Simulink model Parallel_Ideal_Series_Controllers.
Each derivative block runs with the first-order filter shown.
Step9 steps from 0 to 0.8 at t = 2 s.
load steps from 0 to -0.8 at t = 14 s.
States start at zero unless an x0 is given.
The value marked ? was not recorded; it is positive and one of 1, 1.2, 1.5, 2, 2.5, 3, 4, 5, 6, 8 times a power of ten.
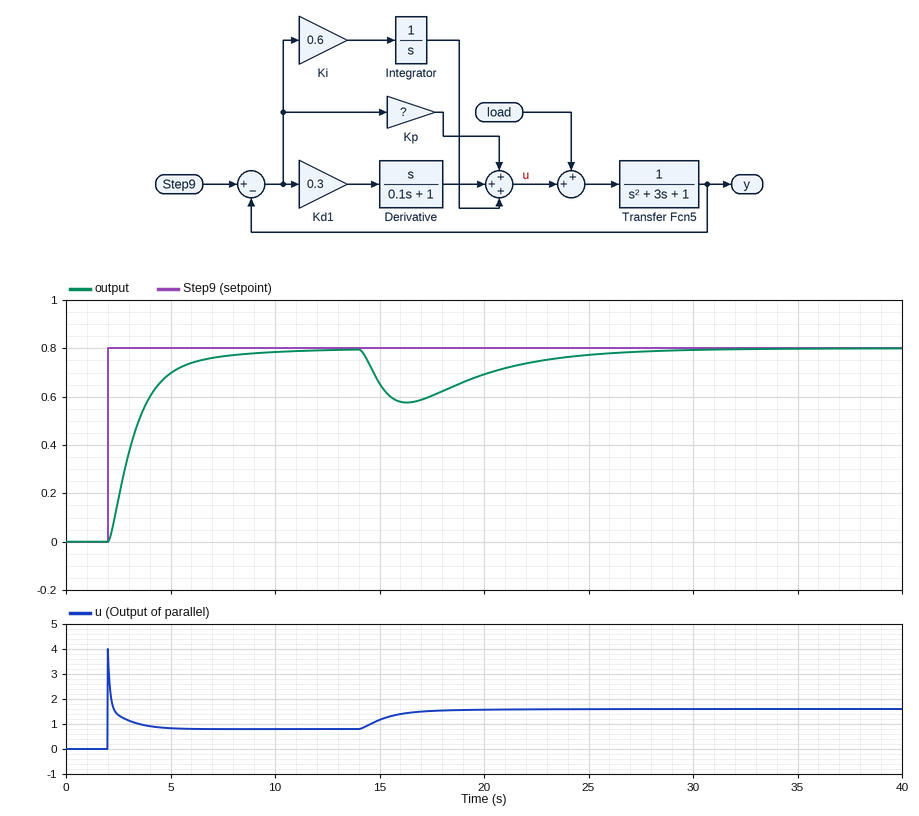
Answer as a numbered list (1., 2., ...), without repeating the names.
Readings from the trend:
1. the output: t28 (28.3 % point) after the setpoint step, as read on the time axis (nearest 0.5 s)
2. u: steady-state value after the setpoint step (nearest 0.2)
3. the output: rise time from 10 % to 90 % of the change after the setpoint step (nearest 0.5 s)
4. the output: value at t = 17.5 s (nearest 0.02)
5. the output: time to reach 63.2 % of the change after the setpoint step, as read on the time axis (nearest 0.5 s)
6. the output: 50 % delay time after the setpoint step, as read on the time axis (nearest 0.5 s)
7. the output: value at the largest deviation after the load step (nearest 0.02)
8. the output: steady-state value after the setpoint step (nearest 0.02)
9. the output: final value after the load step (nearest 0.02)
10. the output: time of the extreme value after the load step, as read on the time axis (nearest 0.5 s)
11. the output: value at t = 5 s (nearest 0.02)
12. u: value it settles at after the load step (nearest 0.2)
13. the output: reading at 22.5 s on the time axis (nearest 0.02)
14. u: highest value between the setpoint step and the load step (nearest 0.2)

1. 2.5 s
2. 0.8
3. 3.0 s
4. 0.60
5. 3.5 s
6. 3.0 s
7. 0.58
8. 0.80
9. 0.80
10. 16.5 s
11. 0.70
12. 1.6
13. 0.74
14. 4.0
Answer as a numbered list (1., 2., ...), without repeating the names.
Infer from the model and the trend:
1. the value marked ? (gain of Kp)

1. 2
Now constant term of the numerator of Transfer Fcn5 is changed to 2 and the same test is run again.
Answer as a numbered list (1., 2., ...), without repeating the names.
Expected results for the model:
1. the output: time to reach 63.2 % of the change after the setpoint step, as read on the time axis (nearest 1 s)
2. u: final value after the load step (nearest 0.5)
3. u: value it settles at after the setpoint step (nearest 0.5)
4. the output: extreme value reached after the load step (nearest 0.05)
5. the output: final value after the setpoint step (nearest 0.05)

1. 3 s
2. 1.0
3. 0.5
4. 0.50
5. 0.80
